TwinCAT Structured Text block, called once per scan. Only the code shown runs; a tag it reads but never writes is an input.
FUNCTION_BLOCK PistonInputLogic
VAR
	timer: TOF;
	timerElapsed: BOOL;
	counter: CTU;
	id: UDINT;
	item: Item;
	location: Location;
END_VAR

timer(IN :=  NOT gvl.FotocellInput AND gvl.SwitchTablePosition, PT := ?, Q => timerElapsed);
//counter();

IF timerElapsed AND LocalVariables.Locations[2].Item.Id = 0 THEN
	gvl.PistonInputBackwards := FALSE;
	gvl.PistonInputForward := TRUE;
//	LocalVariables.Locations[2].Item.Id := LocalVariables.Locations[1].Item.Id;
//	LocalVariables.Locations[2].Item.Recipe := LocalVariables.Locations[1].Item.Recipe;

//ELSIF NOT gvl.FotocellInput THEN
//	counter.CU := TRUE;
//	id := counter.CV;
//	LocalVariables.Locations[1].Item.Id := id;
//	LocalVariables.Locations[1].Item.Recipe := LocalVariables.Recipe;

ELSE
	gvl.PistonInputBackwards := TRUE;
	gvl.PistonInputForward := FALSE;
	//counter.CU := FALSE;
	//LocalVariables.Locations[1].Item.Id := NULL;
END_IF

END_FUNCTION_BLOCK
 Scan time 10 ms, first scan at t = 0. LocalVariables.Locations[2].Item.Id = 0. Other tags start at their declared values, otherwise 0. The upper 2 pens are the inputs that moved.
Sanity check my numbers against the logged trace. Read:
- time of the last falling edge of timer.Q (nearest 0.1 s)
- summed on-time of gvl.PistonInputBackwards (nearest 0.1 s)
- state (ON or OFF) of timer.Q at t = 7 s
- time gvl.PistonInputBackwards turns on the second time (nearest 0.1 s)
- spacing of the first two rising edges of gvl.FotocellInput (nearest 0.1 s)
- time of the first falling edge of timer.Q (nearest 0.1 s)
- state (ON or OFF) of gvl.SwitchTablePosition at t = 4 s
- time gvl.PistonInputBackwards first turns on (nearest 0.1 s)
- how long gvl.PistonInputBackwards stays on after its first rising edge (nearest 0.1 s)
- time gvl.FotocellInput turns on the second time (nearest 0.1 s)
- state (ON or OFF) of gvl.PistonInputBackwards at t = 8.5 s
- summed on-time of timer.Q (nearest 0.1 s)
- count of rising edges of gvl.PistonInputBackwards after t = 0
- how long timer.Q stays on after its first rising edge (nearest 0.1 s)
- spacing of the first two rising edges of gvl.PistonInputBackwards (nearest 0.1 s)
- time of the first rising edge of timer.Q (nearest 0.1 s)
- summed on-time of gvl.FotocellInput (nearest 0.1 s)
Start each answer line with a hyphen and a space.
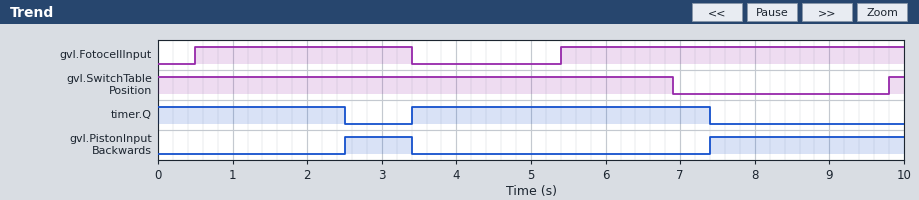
- 7.4 s
- 3.5 s
- ON
- 7.4 s
- 4.9 s
- 2.5 s
- ON
- 2.5 s
- 0.9 s
- 5.4 s
- ON
- 6.5 s
- 2
- 4.0 s
- 4.9 s
- 3.4 s
- 7.5 s
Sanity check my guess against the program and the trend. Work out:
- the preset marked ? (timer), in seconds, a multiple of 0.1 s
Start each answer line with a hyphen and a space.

- 2.0 s
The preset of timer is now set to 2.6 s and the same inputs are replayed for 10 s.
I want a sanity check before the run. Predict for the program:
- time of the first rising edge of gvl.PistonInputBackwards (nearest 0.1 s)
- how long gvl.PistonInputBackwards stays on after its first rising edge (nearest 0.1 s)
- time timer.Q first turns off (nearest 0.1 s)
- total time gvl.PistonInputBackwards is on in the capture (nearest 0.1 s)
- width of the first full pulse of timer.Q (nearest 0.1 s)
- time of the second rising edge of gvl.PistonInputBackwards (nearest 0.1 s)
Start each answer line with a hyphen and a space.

- 3.1 s
- 0.3 s
- 3.1 s
- 2.3 s
- 4.6 s
- 8.0 s
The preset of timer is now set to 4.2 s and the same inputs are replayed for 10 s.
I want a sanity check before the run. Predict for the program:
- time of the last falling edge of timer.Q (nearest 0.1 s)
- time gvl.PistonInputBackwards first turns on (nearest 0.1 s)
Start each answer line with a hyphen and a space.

- 9.6 s
- 9.6 s
